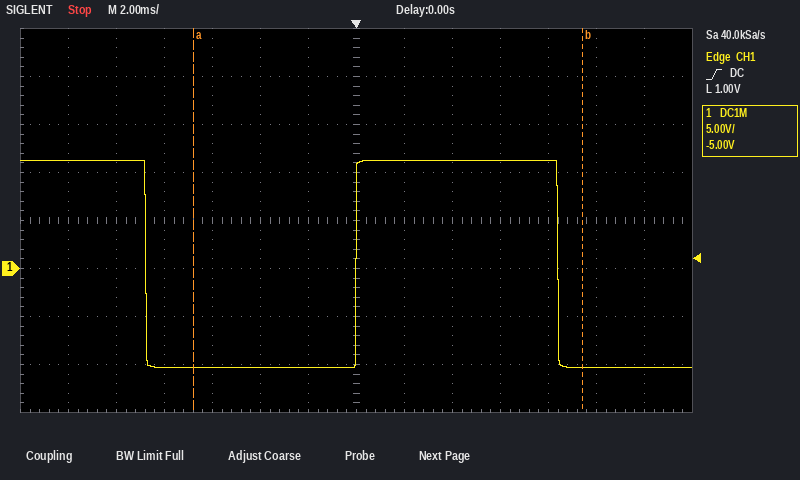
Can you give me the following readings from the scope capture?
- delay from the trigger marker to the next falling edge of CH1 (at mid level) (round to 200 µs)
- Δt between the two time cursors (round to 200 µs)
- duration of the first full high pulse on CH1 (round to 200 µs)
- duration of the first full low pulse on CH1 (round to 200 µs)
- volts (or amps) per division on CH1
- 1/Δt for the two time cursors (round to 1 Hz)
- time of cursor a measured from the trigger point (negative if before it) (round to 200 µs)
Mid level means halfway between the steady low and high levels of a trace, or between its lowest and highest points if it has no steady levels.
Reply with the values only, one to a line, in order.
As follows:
8.4 ms
16.2 ms
8.4 ms
8.8 ms
5 V
62 Hz
-6.8 ms
